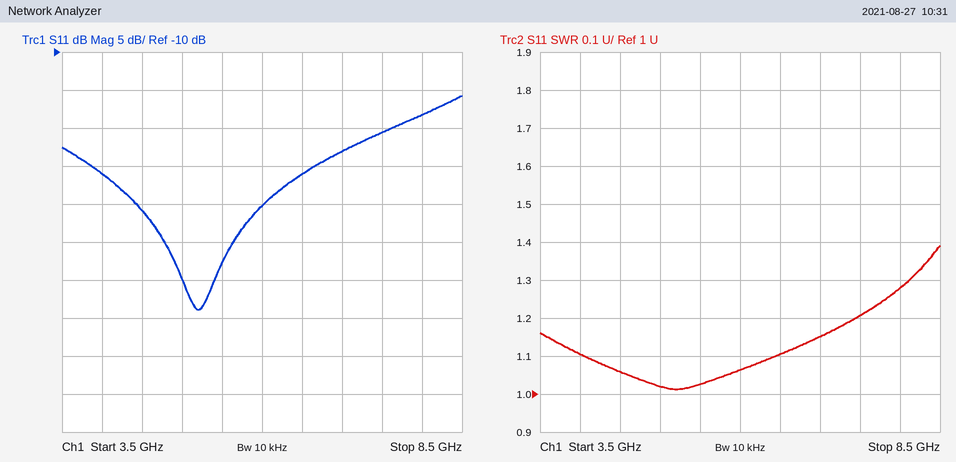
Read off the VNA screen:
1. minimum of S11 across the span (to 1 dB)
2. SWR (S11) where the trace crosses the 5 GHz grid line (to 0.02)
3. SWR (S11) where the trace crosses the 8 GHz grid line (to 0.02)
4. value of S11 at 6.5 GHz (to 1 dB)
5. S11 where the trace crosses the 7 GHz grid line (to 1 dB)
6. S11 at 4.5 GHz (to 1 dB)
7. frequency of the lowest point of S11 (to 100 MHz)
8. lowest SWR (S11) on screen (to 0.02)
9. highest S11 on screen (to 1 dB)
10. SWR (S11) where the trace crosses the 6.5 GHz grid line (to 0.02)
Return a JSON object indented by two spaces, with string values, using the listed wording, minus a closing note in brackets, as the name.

{
  "minimum of S11 across the span": "-44 dB",
  "SWR (S11) where the trace crosses the 5 GHz grid line": "1.02",
  "SWR (S11) where the trace crosses the 8 GHz grid line": "1.28",
  "value of S11 at 6.5 GHz": "-26 dB",
  "S11 where the trace crosses the 7 GHz grid line": "-23 dB",
  "S11 at 4.5 GHz": "-31 dB",
  "frequency of the lowest point of S11": "5.2 GHz",
  "lowest SWR (S11) on screen": "1.02",
  "highest S11 on screen": "-16 dB",
  "SWR (S11) where the trace crosses the 6.5 GHz grid line": "1.10"
}
